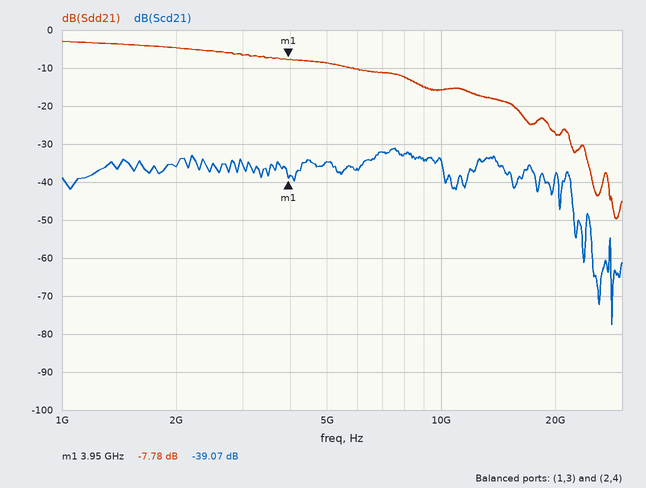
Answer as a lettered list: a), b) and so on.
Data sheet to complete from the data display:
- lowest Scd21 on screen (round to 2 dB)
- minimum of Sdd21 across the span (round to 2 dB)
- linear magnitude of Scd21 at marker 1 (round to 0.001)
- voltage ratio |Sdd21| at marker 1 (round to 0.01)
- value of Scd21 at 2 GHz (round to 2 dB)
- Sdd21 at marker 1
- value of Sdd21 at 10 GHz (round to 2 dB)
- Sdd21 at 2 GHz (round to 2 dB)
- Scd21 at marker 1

a) -78 dB
b) -50 dB
c) 0.011
d) 0.41
e) -36 dB
f) -7.78 dB
g) -16 dB
h) -4 dB
i) -39.07 dB
